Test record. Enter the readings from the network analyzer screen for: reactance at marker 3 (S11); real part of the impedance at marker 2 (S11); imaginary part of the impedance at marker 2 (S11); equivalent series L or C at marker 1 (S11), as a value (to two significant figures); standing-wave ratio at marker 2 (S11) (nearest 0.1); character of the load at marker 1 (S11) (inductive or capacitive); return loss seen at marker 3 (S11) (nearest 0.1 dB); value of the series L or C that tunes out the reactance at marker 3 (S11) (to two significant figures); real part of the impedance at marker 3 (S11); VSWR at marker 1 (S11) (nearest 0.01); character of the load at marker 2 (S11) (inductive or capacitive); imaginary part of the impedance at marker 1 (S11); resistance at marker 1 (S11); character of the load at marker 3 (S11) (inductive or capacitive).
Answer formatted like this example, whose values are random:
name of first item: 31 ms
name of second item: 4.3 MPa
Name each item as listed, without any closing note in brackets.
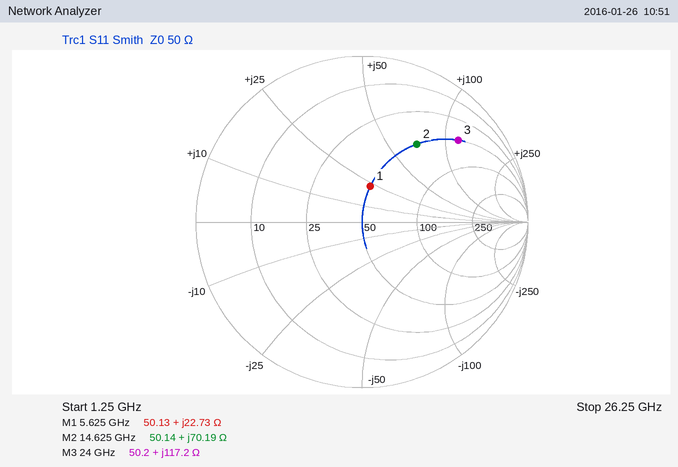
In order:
reactance at marker 3: +117.2 Ω
real part of the impedance at marker 2: 50.14 Ω
imaginary part of the impedance at marker 2: +70.19 Ω
equivalent series L or C at marker 1 (S11), as a value: 640 pH
standing-wave ratio at marker 2 (S11): 3.7
character of the load at marker 1 (S11): inductive
return loss seen at marker 3 (S11): 2.4 dB
value of the series L or C that tunes out the reactance at marker 3 (S11): 57 fF
real part of the impedance at marker 3: 50.2 Ω
VSWR at marker 1 (S11): 1.57
character of the load at marker 2 (S11): inductive
imaginary part of the impedance at marker 1: +22.73 Ω
resistance at marker 1: 50.13 Ω
character of the load at marker 3 (S11): inductive
